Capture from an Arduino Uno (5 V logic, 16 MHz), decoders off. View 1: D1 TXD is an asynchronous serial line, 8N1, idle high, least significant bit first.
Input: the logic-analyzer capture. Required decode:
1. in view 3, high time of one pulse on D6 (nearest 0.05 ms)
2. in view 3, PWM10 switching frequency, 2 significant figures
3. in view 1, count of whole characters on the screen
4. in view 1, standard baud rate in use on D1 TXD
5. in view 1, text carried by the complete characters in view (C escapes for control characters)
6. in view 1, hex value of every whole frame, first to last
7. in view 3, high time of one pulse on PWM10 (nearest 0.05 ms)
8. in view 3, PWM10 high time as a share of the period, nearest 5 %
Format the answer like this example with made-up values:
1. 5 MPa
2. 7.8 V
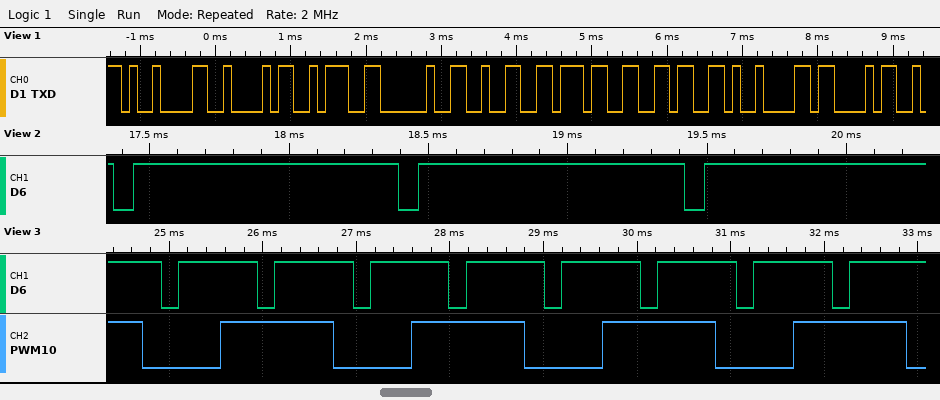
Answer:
1. 0.85 ms
2. 490 Hz
3. 9
4. 9600 baud
5. "\tB: 276\tC"
6. 09 42 3A 20 32 37 36 09 43
7. 1.20 ms
8. 60 %
